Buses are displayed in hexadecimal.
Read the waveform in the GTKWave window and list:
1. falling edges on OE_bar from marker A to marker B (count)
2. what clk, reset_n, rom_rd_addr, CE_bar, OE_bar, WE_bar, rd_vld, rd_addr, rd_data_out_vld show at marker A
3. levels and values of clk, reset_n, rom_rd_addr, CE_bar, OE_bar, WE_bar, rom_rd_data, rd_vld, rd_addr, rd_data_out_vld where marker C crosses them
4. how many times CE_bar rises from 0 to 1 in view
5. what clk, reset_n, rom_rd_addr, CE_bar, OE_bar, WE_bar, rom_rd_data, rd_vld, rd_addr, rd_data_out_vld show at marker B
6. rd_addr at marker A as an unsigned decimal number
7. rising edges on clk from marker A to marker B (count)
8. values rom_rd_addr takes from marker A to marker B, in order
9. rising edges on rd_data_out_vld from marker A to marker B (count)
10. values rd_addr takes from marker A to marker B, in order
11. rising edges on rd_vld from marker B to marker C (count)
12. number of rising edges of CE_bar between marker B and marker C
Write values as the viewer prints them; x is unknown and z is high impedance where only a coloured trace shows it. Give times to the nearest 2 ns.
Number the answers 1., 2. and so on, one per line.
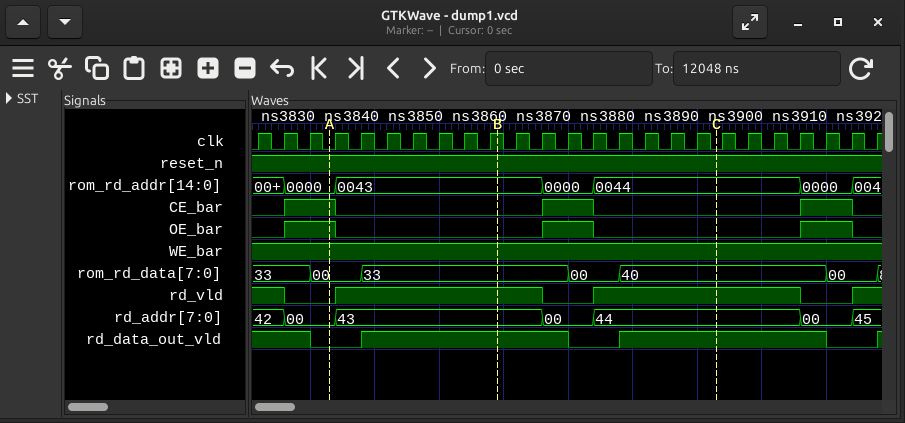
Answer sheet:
1. 1
2. clk=0, reset_n=1, rom_rd_addr=0000, CE_bar=1, OE_bar=1, WE_bar=1, rd_vld=0, rd_addr=00, rd_data_out_vld=0
3. clk=0, reset_n=1, rom_rd_addr=0044, CE_bar=0, OE_bar=0, WE_bar=1, rom_rd_data=40, rd_vld=1, rd_addr=44, rd_data_out_vld=1
4. 3
5. clk=1, reset_n=1, rom_rd_addr=0043, CE_bar=0, OE_bar=0, WE_bar=1, rom_rd_data=33, rd_vld=1, rd_addr=43, rd_data_out_vld=1
6. 0
7. 7
8. 0000, 0043
9. 1
10. 00, 43
11. 1
12. 1
